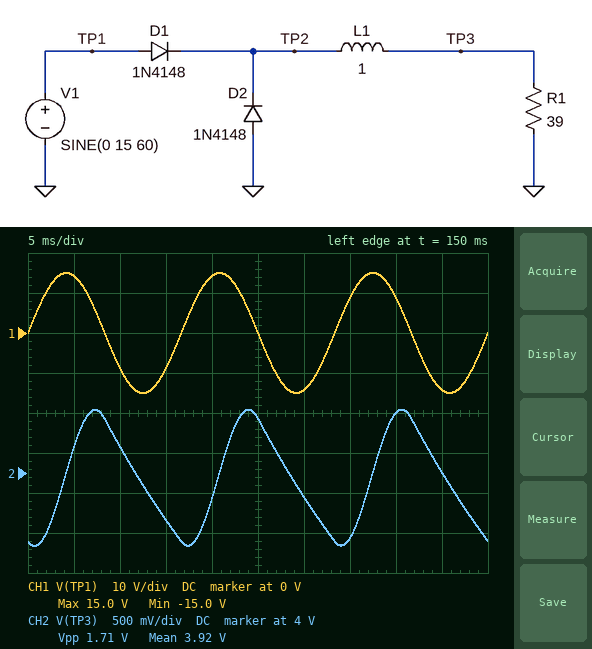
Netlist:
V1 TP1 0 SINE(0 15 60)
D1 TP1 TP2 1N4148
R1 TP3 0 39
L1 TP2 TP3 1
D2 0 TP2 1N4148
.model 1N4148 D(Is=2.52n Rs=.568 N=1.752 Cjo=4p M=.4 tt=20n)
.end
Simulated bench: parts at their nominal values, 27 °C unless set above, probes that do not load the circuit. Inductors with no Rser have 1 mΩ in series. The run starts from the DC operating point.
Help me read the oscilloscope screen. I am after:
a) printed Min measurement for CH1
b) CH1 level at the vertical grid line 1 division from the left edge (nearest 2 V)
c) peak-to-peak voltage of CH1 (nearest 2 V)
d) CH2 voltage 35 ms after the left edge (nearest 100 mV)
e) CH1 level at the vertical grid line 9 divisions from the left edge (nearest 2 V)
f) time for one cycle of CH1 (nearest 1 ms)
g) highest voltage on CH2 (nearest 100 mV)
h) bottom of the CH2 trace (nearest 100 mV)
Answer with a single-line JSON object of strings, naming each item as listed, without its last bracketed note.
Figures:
{"printed Min measurement for CH1": "-15.0 V", "CH1 level at the vertical grid line 1 division from the left edge": "14 V", "peak-to-peak voltage of CH1": "30 V", "CH2 voltage 35 ms after the left edge": "3.2 V", "CH1 level at the vertical grid line 9 divisions from the left edge": "-14 V", "time for one cycle of CH1": "17 ms", "highest voltage on CH2": "4.8 V", "bottom of the CH2 trace": "3.1 V"}
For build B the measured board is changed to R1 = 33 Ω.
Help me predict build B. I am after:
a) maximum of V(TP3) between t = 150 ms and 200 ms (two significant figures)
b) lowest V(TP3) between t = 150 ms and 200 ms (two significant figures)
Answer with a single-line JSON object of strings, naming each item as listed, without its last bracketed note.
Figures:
{"maximum of V(TP3) between t = 150 ms and 200 ms": "4.6 V", "lowest V(TP3) between t = 150 ms and 200 ms": "3.2 V"}
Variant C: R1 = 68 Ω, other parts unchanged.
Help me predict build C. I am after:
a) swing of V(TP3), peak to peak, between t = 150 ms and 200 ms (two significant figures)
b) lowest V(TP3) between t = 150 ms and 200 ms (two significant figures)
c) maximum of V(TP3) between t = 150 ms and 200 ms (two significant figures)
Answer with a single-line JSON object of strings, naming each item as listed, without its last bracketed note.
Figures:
{"swing of V(TP3), peak to peak, between t = 150 ms and 200 ms": "2.9 V", "lowest V(TP3) between t = 150 ms and 200 ms": "2.6 V", "maximum of V(TP3) between t = 150 ms and 200 ms": "5.5 V"}
